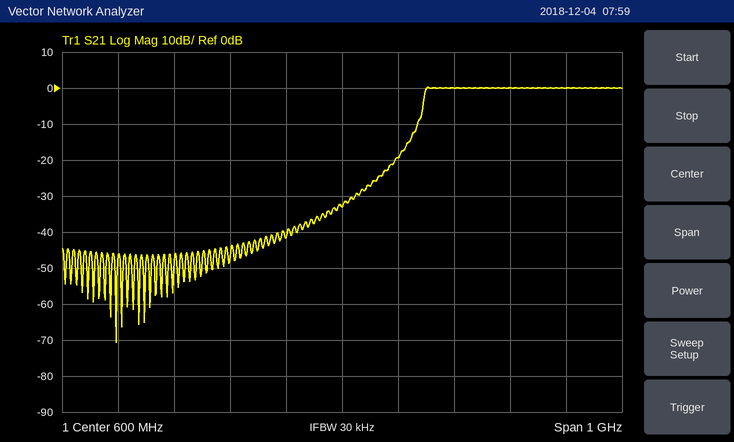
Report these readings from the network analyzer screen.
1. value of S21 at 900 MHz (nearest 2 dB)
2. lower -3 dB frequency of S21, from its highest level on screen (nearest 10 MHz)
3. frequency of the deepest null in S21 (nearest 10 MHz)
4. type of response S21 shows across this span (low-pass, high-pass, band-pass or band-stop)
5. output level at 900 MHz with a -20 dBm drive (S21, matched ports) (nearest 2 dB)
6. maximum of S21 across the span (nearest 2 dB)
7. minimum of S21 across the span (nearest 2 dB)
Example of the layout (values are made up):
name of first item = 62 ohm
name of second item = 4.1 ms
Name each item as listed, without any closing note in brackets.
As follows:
value of S21 at 900 MHz = 0 dB
lower -3 dB frequency of S21, from its highest level on screen = 750 MHz
frequency of the deepest null in S21 = 200 MHz
type of response S21 shows across this span = high-pass
output level at 900 MHz with a -20 dBm drive (S21, matched ports) = -20 dBm
maximum of S21 across the span = 0 dB
minimum of S21 across the span = -70 dB
